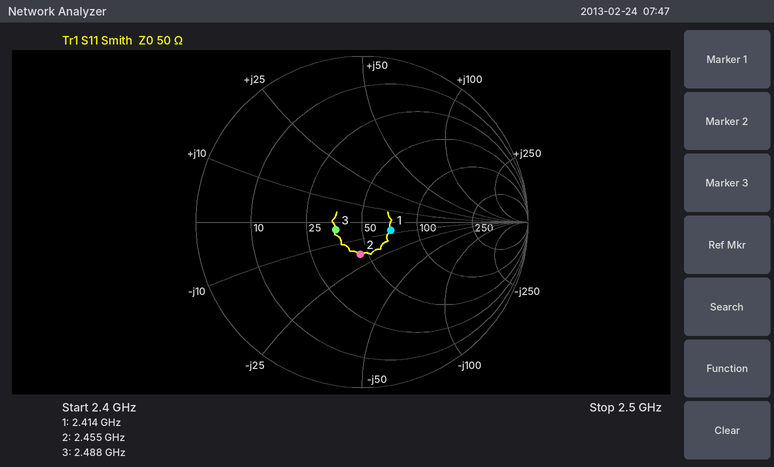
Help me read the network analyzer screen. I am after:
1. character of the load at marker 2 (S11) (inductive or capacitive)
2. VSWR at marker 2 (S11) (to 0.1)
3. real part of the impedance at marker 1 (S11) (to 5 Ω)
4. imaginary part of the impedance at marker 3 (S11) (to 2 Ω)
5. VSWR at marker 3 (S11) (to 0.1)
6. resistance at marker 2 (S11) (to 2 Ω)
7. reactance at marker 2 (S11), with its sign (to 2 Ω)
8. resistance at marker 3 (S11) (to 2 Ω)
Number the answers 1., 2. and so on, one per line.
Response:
1. capacitive
2. 1.5
3. 70 Ω
4. -4 Ω
5. 1.4
6. 46 Ω
7. -18 Ω
8. 36 Ω
